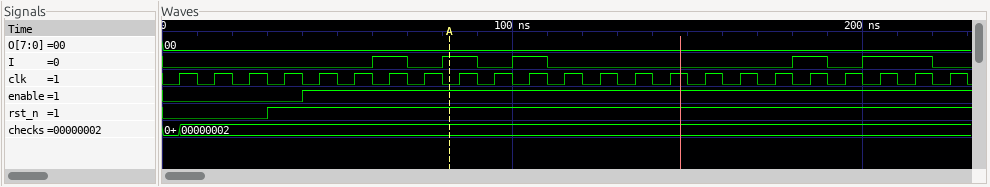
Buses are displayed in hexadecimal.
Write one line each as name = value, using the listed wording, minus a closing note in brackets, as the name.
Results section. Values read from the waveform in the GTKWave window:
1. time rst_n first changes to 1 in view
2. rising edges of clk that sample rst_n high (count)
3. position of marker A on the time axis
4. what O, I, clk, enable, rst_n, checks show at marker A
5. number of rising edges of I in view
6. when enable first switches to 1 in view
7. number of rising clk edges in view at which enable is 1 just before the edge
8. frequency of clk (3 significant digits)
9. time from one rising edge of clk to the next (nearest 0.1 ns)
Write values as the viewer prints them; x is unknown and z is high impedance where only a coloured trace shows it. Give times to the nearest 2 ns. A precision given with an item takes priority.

time rst_n first changes to 1 in view = 30 ns
rising edges of clk that sample rst_n high = 20
position of marker A on the time axis = 82 ns
what O, I, clk, enable, rst_n, checks show at marker A = O=00, I=1, clk=0, enable=1, rst_n=1, checks=00000002
number of rising edges of I in view = 5
when enable first switches to 1 in view = 40 ns
number of rising clk edges in view at which enable is 1 just before the edge = 19
frequency of clk = 100 MHz
time from one rising edge of clk to the next = 10 ns
